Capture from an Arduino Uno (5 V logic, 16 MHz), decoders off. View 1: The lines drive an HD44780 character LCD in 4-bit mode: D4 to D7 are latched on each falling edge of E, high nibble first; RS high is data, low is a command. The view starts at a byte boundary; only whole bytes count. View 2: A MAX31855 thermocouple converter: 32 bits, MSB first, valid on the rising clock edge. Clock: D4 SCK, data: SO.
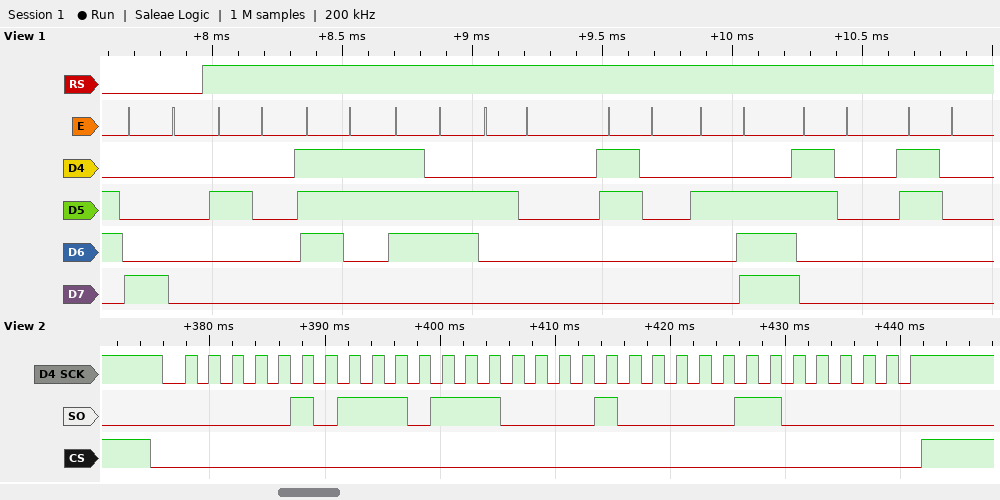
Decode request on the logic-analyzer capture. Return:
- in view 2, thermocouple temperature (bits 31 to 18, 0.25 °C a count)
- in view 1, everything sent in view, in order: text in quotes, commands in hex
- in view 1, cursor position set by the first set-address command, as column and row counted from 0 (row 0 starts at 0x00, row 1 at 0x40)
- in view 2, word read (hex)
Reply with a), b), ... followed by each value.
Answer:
a) 93.75 °C
b) 0x80 " sv 0.00"
c) column 0, row 0
d) 0x05DC20C0
